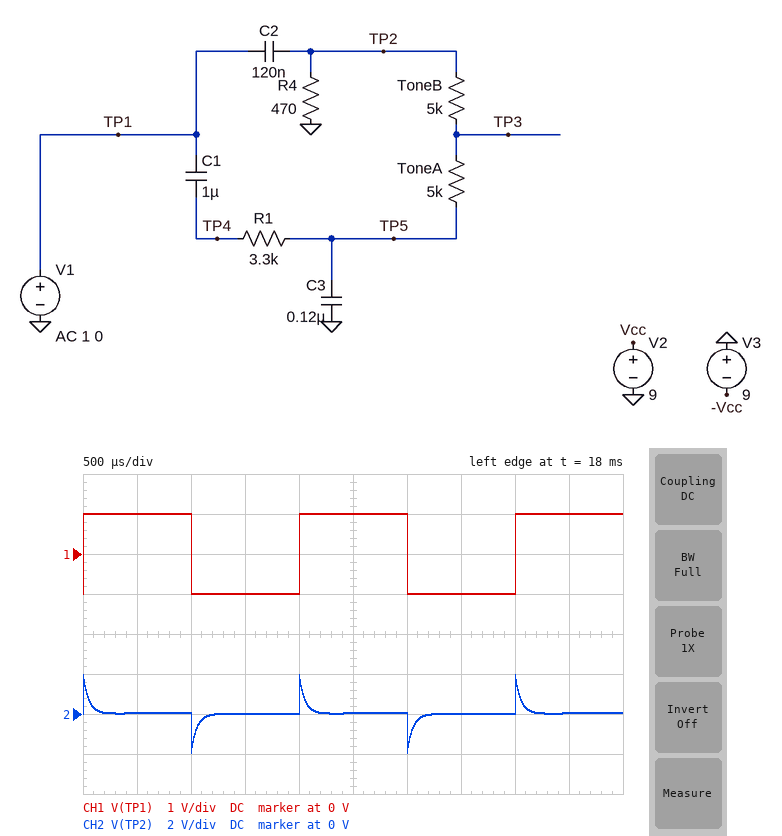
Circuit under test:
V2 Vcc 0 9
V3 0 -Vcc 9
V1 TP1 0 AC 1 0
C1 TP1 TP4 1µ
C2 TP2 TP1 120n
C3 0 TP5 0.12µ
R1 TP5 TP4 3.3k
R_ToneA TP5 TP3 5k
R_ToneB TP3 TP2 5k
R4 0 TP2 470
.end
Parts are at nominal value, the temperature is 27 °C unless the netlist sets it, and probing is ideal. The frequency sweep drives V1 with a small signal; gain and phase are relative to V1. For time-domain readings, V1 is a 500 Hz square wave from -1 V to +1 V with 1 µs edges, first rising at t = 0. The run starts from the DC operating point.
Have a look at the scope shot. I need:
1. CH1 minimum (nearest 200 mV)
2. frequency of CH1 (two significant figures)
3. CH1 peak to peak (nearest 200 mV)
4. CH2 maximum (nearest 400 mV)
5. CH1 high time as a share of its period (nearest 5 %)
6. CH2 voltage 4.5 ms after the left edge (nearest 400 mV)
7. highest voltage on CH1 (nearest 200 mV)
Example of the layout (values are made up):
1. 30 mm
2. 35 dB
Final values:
1. -1.0 V
2. 500 Hz
3. 2.0 V
4. 2.0 V
5. 50 %
6. 0 V
7. 1.0 V
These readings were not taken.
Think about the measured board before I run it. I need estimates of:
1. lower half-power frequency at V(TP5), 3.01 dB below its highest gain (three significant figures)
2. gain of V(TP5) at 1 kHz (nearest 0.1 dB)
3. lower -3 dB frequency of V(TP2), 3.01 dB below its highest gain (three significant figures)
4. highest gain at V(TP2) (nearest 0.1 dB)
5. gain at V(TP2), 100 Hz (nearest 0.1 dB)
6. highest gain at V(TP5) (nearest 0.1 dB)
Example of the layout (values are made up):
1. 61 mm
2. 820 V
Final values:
1. 10.4 Hz
2. -8.8 dB
3. 2.99 kHz
4. 0 dB
5. -27.0 dB
6. -3.1 dB
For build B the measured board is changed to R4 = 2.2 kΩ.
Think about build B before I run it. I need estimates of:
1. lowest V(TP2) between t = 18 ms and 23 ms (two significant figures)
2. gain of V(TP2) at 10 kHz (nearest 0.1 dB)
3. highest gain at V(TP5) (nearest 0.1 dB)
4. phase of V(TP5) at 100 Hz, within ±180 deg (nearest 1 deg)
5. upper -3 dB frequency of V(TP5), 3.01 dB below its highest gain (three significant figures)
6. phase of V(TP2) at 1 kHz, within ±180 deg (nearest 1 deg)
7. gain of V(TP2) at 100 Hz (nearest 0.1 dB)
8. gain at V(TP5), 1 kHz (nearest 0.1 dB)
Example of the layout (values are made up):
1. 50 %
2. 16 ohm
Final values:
1. -1.8 V
2. 0 dB
3. -2.7 dB
4. -3 deg
5. 708 Hz
6. 34 deg
7. -14.7 dB
8. -7.4 dB
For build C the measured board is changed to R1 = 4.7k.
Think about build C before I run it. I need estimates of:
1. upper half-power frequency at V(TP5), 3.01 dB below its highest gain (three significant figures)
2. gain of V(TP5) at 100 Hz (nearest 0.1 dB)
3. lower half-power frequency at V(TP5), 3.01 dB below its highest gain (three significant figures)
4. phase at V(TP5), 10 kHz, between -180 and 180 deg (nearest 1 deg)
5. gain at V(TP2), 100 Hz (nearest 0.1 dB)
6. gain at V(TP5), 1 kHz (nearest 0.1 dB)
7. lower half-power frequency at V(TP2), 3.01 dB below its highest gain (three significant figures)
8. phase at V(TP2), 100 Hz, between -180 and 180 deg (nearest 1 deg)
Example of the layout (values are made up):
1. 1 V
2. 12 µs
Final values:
1. 463 Hz
2. -3.9 dB
3. 9.49 Hz
4. -82 deg
5. -27.6 dB
6. -11.2 dB
7. 2.98 kHz
8. 45 deg
